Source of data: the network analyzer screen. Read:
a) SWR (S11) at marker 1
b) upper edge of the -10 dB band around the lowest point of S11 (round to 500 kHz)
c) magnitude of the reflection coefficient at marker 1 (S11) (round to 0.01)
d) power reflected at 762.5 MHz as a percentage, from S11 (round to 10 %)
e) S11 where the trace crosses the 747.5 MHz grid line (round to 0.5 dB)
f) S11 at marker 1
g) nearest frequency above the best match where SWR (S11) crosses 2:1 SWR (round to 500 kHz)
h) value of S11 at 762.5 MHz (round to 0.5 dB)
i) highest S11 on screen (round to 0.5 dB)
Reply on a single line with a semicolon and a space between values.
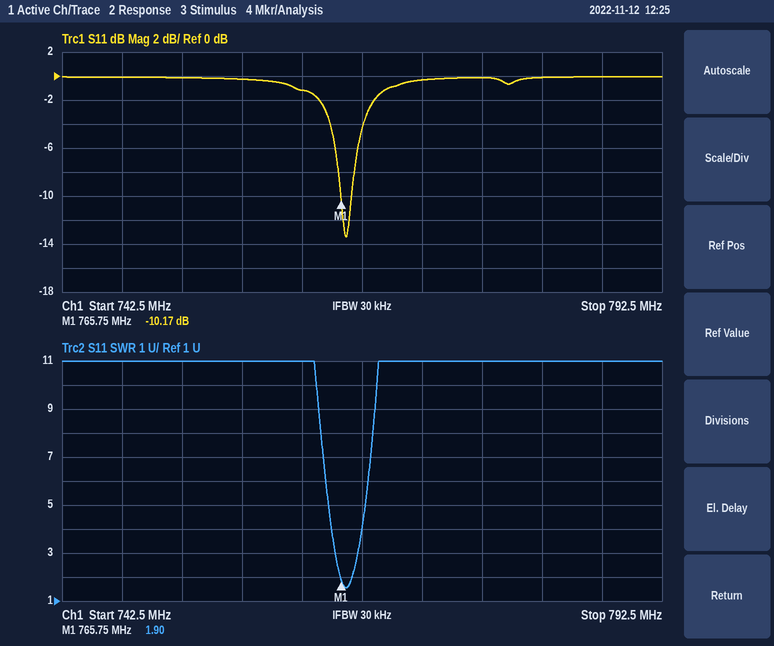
1.90; 766.5 MHz; 0.31; 80 %; 0.0 dB; -10.17 dB; 766.5 MHz; -1.0 dB; 0.0 dB
